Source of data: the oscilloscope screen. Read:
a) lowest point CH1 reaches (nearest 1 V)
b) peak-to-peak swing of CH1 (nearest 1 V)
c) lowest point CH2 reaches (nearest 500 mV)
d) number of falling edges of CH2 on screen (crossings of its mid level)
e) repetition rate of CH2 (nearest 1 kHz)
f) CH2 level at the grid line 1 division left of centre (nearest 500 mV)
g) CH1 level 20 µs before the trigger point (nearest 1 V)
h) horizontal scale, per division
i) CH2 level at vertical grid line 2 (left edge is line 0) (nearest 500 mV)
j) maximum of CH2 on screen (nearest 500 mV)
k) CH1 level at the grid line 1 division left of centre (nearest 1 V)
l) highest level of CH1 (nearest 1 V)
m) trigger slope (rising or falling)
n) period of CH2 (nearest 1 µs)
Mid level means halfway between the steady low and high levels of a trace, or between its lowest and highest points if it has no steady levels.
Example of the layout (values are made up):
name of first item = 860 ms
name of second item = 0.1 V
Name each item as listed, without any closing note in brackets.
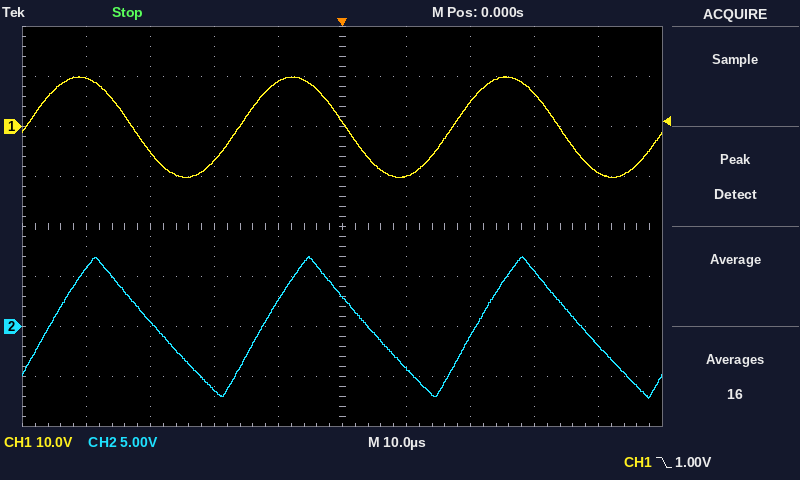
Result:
lowest point CH1 reaches = -10 V
peak-to-peak swing of CH1 = 20 V
lowest point CH2 reaches = -7.0 V
number of falling edges of CH2 on screen = 3
repetition rate of CH2 = 30 kHz
CH2 level at the grid line 1 division left of centre = 2.5 V
CH1 level 20 µs before the trigger point = -7 V
horizontal scale, per division = 10 µs
CH2 level at vertical grid line 2 (left edge is line 0) = 500 mV
maximum of CH2 on screen = 7.0 V
CH1 level at the grid line 1 division left of centre = 9 V
highest level of CH1 = 10 V
trigger slope = falling
period of CH2 = 33 µs
